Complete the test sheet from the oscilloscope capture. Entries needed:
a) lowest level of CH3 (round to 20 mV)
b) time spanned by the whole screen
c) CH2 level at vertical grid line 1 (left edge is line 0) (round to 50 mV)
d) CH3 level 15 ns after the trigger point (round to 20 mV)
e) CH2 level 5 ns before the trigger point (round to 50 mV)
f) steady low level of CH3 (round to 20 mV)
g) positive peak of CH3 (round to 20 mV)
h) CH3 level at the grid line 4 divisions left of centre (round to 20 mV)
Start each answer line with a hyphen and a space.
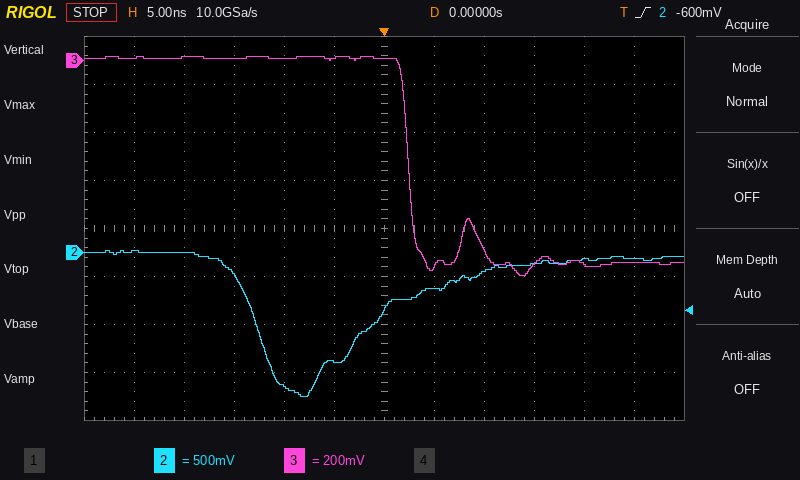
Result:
- -900 mV
- 60 ns
- 0 mV
- -840 mV
- -1.15 V
- -840 mV
- 20 mV
- 20 mV
